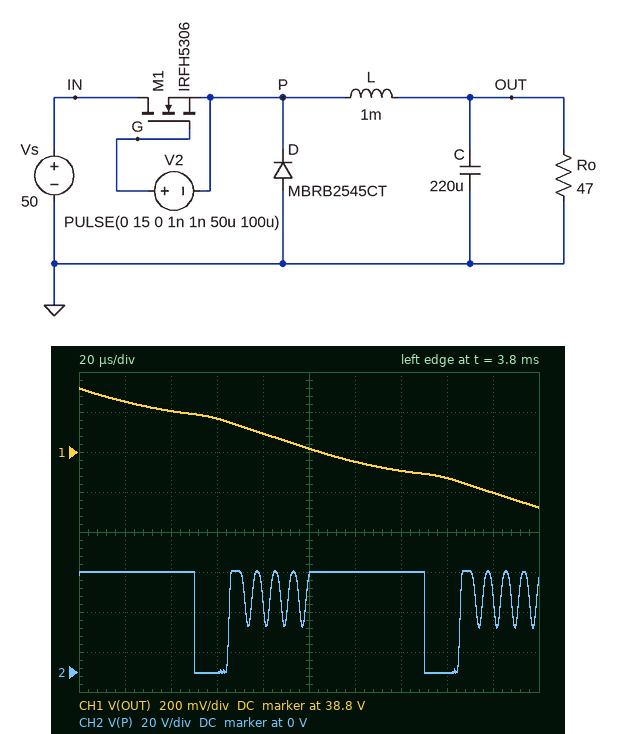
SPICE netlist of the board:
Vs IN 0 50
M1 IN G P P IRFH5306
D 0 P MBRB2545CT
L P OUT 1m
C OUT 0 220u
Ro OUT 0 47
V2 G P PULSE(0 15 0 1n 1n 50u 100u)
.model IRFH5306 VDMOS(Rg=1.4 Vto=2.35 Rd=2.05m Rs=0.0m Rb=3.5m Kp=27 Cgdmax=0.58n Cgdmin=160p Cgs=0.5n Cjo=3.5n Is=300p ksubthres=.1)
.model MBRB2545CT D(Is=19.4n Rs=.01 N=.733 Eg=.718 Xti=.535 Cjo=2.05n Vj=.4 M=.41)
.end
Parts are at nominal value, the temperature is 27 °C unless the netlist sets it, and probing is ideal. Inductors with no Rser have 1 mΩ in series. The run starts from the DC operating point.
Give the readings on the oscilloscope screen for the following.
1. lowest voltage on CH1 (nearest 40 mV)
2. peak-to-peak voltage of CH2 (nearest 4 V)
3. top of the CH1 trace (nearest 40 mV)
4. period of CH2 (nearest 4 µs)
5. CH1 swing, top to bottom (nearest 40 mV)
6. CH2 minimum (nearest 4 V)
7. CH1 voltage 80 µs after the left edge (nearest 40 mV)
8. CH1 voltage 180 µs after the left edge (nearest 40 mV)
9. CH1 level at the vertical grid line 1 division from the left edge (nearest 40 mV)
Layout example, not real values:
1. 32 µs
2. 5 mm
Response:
1. 38.52 V
2. 52 V
3. 39.12 V
4. 100 µs
5. 600 mV
6. 0 V
7. 38.88 V
8. 38.60 V
9. 39.04 V
